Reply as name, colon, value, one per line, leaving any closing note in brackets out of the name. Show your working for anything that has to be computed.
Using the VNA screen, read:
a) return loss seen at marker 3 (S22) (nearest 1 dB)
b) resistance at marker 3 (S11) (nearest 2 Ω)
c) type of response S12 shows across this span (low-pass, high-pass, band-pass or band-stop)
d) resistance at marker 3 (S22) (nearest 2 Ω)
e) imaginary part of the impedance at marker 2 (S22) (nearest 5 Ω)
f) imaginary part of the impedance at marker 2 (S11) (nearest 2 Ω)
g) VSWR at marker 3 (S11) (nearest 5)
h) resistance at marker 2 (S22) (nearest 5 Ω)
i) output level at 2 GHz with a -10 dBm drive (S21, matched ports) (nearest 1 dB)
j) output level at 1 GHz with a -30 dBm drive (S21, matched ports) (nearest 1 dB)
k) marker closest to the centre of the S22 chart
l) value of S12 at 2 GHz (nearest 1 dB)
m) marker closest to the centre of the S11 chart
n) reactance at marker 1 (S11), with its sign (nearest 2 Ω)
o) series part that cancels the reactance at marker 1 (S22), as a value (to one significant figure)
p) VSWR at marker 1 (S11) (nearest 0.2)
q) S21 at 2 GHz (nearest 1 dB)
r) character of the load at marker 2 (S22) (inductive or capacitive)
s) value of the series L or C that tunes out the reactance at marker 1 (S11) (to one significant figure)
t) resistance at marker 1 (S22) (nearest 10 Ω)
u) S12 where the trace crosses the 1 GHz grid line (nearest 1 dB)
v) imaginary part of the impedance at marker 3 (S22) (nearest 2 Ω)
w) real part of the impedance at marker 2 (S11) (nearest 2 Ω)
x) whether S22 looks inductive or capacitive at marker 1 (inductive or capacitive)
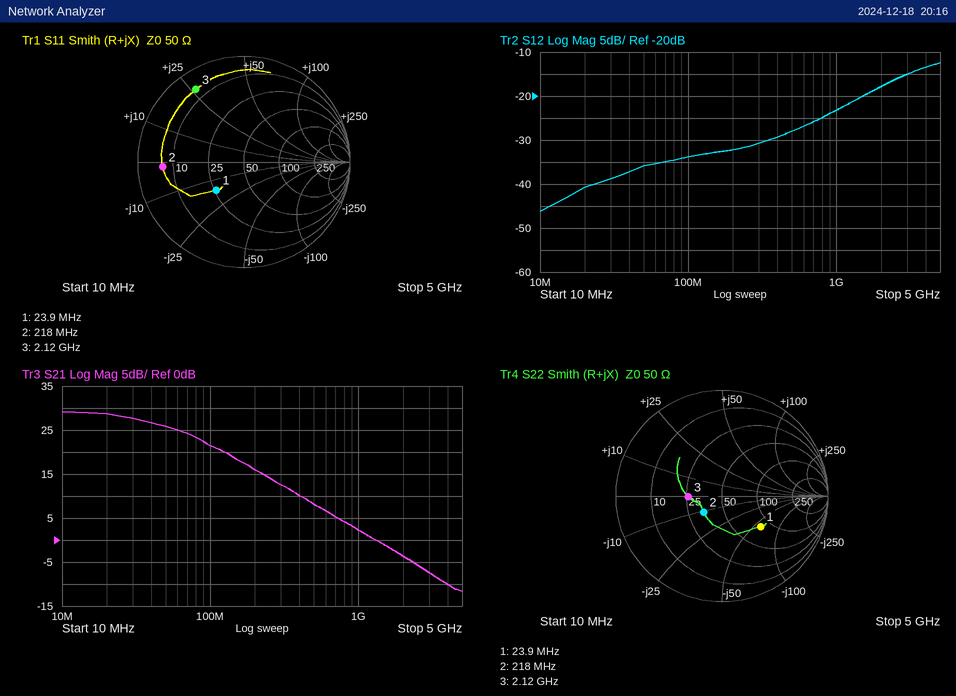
return loss seen at marker 3 (S22): 10 dB
resistance at marker 3 (S11): 6 Ω
type of response S12 shows across this span: high-pass
resistance at marker 3 (S22): 26 Ω
imaginary part of the impedance at marker 2 (S22): -10 Ω
imaginary part of the impedance at marker 2 (S11): -2 Ω
VSWR at marker 3 (S11): 10
resistance at marker 2 (S22): 35 Ω
output level at 2 GHz with a -10 dBm drive (S21, matched ports): -10 dBm + (-4 dB) = -14 dBm
output level at 1 GHz with a -30 dBm drive (S21, matched ports): -30 dBm + (2 dB) = -28 dBm
marker closest to the centre of the S22 chart: marker 2
value of S12 at 2 GHz: -18 dB
marker closest to the centre of the S11 chart: marker 1
reactance at marker 1 (S11), with its sign: -16 Ω
series part that cancels the reactance at marker 1 (S22), as a value: L = 60 Ω/(2π × 23.9 MHz) ≈ 400 nH
VSWR at marker 1 (S11): 2.2
S21 at 2 GHz: -4 dB
character of the load at marker 2 (S22): capacitive
value of the series L or C that tunes out the reactance at marker 1 (S11): L = 16 Ω/(2π × 23.9 MHz) ≈ 107 nH, so 100 nH to one significant figure
resistance at marker 1 (S22): 80 Ω
S12 where the trace crosses the 1 GHz grid line: -23 dB
imaginary part of the impedance at marker 3 (S22): 0 Ω
real part of the impedance at marker 2 (S11): 6 Ω
whether S22 looks inductive or capacitive at marker 1: capacitive
